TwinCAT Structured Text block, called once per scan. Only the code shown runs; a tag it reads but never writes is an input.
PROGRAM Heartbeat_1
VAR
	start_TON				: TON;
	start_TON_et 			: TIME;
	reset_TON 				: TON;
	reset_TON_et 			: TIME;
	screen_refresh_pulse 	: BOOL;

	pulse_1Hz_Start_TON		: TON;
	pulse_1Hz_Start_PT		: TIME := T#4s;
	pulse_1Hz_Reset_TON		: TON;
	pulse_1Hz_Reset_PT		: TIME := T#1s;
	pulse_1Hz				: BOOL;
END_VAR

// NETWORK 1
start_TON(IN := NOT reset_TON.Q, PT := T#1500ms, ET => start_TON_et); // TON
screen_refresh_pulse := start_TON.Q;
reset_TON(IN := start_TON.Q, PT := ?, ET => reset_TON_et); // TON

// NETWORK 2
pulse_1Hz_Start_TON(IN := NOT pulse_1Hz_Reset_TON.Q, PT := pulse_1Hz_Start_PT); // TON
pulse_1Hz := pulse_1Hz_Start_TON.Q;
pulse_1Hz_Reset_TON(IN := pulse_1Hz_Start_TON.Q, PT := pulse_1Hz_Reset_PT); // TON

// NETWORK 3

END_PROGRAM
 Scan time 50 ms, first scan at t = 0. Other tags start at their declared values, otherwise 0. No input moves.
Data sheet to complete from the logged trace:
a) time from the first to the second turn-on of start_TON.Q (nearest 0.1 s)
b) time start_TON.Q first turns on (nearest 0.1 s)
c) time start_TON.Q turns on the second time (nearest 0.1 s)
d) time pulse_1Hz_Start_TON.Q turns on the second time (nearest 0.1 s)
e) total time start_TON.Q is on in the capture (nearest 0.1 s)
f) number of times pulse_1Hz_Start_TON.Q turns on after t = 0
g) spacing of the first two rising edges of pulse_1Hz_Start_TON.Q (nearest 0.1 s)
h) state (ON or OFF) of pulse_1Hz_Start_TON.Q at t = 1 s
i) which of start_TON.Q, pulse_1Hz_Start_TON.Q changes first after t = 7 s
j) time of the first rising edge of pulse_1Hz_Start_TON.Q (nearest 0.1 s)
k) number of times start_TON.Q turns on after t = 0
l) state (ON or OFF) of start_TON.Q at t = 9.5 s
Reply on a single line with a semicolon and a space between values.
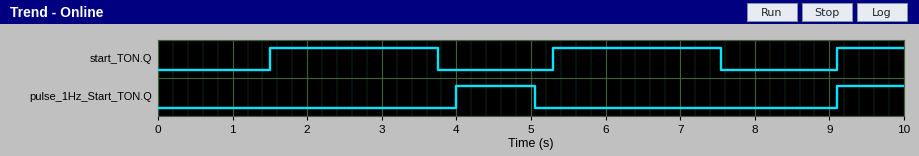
3.8 s; 1.5 s; 5.3 s; 9.1 s; 5.4 s; 2; 5.1 s; OFF; start_TON.Q; 4.0 s; 3; ON
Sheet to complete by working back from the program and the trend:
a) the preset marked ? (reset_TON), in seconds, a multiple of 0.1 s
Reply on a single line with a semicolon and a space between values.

2.2 s
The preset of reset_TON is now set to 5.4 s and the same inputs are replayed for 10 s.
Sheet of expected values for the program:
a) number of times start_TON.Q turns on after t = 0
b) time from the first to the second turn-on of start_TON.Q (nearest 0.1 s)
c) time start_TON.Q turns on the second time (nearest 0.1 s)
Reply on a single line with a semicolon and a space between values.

2; 7.0 s; 8.5 s
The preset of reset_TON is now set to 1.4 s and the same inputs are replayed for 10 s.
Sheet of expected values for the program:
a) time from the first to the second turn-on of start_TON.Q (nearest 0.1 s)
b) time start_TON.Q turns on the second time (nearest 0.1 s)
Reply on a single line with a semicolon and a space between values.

3.0 s; 4.5 s
